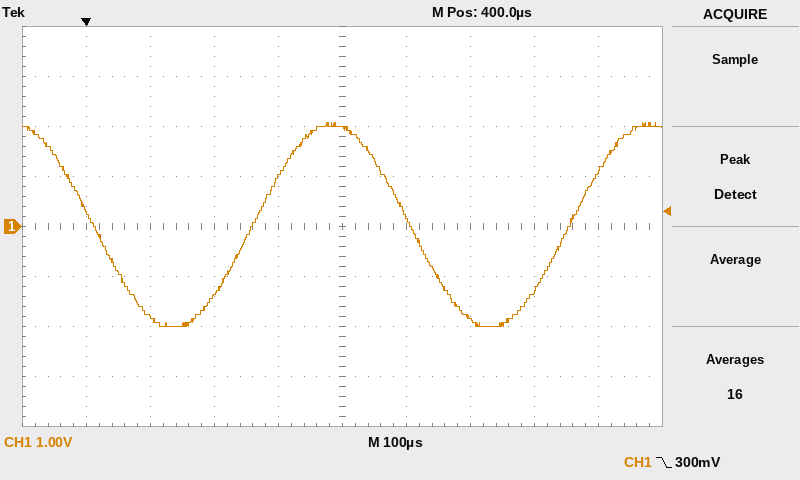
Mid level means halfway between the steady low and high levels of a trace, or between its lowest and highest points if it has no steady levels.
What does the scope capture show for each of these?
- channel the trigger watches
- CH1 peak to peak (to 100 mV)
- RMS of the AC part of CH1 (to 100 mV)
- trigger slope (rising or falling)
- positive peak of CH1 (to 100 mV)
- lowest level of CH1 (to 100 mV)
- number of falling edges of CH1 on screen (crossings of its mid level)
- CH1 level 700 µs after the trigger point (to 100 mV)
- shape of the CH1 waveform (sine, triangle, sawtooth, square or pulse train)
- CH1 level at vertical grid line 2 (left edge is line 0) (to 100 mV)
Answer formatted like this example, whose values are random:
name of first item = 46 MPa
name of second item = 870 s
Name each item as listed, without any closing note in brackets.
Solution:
channel the trigger watches = CH1
CH1 peak to peak = 4.1 V
RMS of the AC part of CH1 = 1.4 V
trigger slope = falling
positive peak of CH1 = 2.1 V
lowest level of CH1 = -2.0 V
number of falling edges of CH1 on screen = 2
CH1 level 700 µs after the trigger point = -1.3 V
shape of the CH1 waveform = sine
CH1 level at vertical grid line 2 (left edge is line 0) = -1.8 V
